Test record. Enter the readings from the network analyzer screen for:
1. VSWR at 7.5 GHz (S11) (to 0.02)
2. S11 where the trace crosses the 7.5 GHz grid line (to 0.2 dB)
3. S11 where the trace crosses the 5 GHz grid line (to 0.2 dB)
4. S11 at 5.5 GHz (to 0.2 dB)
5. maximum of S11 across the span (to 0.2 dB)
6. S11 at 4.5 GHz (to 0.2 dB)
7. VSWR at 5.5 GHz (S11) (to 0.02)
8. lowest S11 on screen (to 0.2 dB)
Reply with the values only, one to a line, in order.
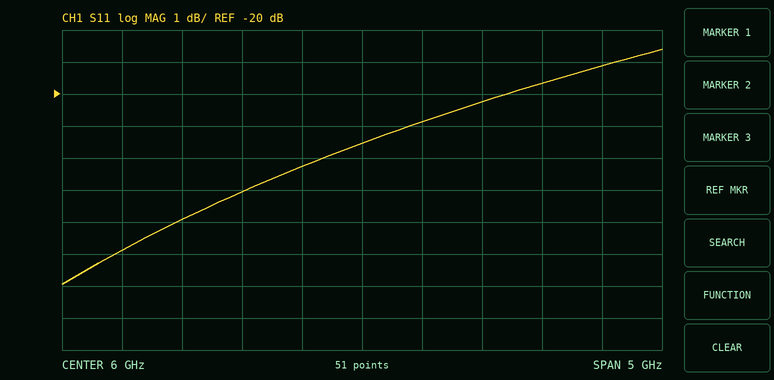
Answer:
1.24
-19.6 dB
-23.0 dB
-22.2 dB
-18.6 dB
-24.0 dB
1.16
-26.0 dB
